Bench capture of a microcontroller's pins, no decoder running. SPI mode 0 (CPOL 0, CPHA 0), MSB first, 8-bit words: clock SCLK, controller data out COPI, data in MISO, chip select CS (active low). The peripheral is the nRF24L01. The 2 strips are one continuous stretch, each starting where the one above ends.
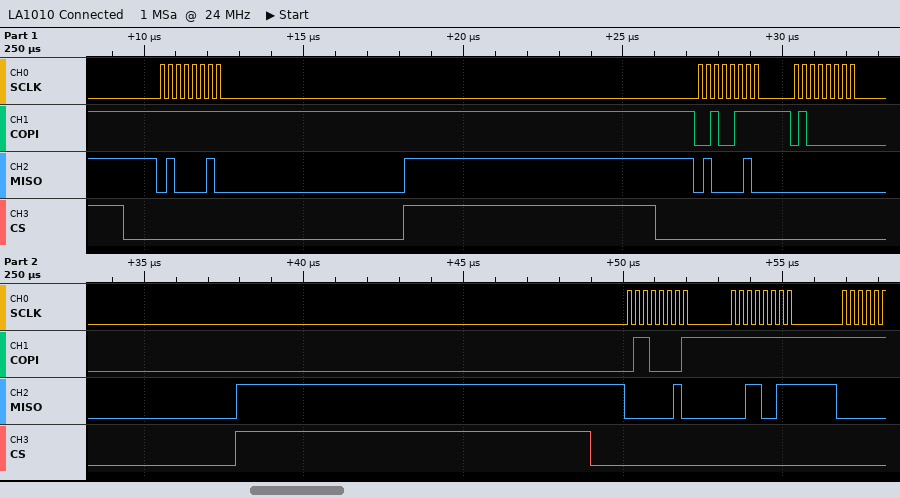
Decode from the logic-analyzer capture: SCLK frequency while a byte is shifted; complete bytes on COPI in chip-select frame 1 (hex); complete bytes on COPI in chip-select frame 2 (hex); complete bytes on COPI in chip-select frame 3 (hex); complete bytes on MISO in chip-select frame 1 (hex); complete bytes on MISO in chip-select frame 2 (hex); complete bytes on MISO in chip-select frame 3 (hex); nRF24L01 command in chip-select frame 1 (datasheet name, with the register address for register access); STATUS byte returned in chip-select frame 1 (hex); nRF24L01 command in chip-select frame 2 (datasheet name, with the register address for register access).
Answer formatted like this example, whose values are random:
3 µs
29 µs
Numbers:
4 MHz
FF
27 40
61 FF
42
42 00
02 33
NOP
0x42
W_REGISTER 0x07
